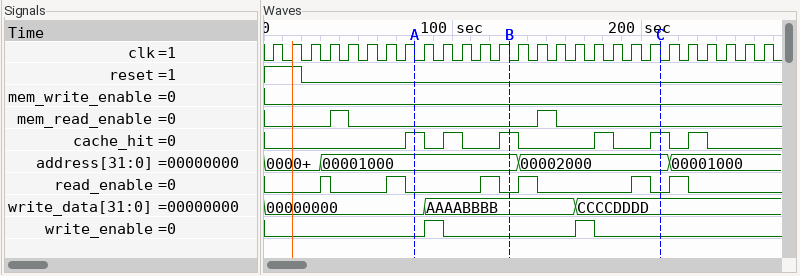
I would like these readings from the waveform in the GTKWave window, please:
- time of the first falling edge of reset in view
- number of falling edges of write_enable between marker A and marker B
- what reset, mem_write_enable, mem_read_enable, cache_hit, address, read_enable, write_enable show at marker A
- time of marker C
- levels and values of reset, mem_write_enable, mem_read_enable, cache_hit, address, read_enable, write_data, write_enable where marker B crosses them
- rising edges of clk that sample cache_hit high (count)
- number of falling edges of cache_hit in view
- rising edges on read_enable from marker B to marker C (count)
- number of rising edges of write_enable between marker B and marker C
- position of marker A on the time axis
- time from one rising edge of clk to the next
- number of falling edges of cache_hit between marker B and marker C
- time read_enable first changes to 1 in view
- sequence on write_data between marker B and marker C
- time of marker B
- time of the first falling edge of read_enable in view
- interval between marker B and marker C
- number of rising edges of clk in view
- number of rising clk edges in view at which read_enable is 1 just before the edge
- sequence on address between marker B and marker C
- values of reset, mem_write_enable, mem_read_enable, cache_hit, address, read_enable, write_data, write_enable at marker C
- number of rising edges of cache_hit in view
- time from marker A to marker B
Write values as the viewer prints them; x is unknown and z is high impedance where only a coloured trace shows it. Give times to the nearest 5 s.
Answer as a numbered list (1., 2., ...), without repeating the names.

1. 20 s
2. 1
3. reset=0, mem_write_enable=0, mem_read_enable=0, cache_hit=1, address=00001000, read_enable=0, write_enable=0
4. 210 s
5. reset=0, mem_write_enable=0, mem_read_enable=0, cache_hit=1, address=00001000, read_enable=0, write_data=AAAABBBB, write_enable=0
6. 6
7. 6
8. 2
9. 1
10. 80 s
11. 10 s
12. 2
13. 30 s
14. AAAABBBB, CCCCDDDD
15. 130 s
16. 35 s
17. 80 s
18. 27
19. 6
20. 00001000, 00002000
21. reset=0, mem_write_enable=0, mem_read_enable=0, cache_hit=1, address=00002000, read_enable=0, write_data=CCCCDDDD, write_enable=0
22. 6
23. 50 s
